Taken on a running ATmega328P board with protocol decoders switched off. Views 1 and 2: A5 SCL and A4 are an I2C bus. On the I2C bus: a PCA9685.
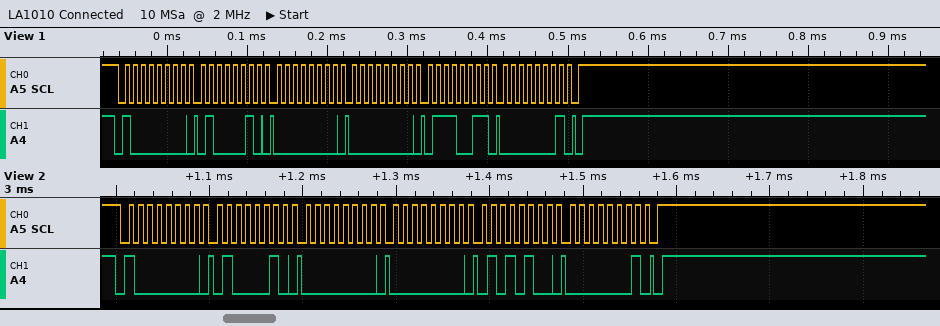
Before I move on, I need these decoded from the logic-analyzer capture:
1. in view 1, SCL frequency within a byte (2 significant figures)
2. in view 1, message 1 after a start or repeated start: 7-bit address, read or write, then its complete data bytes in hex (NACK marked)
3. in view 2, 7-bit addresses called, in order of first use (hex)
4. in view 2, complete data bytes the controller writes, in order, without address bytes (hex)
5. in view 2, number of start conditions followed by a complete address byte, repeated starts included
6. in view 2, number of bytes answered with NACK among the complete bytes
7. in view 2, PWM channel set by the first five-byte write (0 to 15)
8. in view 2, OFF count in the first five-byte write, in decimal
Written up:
100 kHz
0x40 write: 42 00 00 73 01
0x40
42 00 00 54 01
1
0
15
340
